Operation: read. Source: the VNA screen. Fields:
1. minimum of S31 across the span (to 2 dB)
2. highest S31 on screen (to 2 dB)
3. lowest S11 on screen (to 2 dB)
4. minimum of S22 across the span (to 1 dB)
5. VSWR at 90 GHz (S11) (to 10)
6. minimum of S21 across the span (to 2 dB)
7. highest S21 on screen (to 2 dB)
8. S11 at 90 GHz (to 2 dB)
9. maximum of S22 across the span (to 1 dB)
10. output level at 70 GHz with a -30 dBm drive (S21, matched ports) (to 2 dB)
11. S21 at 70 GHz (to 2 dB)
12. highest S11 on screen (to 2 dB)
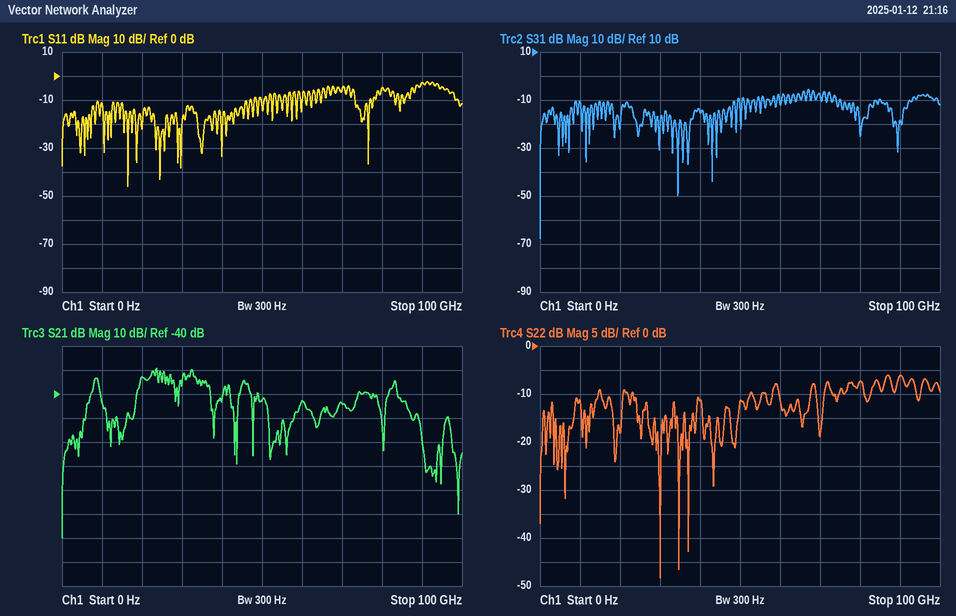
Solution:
-68 dB
-6 dB
-46 dB
-48 dB
10
-100 dB
-30 dB
-2 dB
-6 dB
-74 dBm
-44 dB
-2 dB
